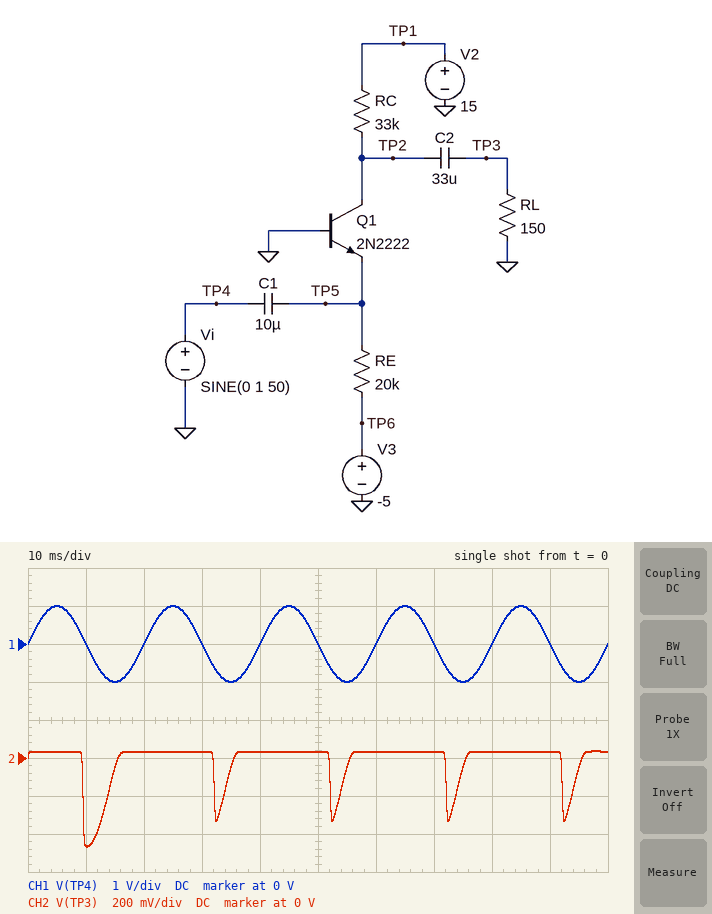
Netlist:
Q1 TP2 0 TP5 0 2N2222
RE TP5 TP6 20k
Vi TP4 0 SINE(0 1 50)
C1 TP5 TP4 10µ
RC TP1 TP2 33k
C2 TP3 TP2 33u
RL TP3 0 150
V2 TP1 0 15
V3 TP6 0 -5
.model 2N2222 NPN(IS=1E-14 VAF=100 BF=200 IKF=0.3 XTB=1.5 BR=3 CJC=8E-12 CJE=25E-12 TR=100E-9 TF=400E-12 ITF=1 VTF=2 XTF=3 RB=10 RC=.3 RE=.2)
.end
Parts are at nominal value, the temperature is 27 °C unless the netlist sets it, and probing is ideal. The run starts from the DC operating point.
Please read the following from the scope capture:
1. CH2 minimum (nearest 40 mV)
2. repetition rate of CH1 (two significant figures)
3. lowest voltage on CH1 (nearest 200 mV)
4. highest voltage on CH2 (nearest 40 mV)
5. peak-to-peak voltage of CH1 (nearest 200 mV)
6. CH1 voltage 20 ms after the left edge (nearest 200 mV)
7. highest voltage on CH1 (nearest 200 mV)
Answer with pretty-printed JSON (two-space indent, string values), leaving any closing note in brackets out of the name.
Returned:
{
  "CH2 minimum": "-480 mV",
  "repetition rate of CH1": "50 Hz",
  "lowest voltage on CH1": "-1.0 V",
  "highest voltage on CH2": "40 mV",
  "peak-to-peak voltage of CH1": "2.0 V",
  "CH1 voltage 20 ms after the left edge": "0 V",
  "highest voltage on CH1": "1.0 V"
}
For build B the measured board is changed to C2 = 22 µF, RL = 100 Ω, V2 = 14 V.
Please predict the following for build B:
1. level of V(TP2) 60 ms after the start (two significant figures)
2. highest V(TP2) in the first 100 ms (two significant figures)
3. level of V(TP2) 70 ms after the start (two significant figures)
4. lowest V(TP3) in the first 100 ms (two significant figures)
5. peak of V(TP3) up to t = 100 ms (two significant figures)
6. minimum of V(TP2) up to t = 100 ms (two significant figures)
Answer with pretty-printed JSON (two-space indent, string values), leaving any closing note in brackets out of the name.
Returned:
{
  "level of V(TP2) 60 ms after the start": "6.4 V",
  "highest V(TP2) in the first 100 ms": "6.9 V",
  "level of V(TP2) 70 ms after the start": "6.5 V",
  "lowest V(TP3) in the first 100 ms": "-310 mV",
  "peak of V(TP3) up to t = 100 ms": "23 mV",
  "minimum of V(TP2) up to t = 100 ms": "6.2 V"
}
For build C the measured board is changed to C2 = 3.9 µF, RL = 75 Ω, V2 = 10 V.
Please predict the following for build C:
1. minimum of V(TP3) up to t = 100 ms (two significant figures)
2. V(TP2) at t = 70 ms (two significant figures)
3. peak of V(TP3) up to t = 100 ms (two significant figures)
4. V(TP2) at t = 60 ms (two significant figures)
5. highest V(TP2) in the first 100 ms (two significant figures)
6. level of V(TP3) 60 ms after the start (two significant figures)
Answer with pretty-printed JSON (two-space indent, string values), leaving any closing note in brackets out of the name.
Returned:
{
  "minimum of V(TP3) up to t = 100 ms": "-230 mV",
  "V(TP2) at t = 70 ms": "1.5 V",
  "peak of V(TP3) up to t = 100 ms": "22 mV",
  "V(TP2) at t = 60 ms": "800 mV",
  "highest V(TP2) in the first 100 ms": "3.3 V",
  "level of V(TP3) 60 ms after the start": "21 mV"
}
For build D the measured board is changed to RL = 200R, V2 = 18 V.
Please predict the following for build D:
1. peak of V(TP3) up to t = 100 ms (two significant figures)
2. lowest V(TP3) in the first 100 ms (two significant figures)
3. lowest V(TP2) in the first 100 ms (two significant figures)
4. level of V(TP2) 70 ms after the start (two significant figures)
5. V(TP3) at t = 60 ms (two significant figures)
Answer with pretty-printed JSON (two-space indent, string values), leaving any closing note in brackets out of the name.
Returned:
{
  "peak of V(TP3) up to t = 100 ms": "46 mV",
  "lowest V(TP3) in the first 100 ms": "-620 mV",
  "lowest V(TP2) in the first 100 ms": "10 V",
  "level of V(TP2) 70 ms after the start": "11 V",
  "V(TP3) at t = 60 ms": "45 mV"
}
